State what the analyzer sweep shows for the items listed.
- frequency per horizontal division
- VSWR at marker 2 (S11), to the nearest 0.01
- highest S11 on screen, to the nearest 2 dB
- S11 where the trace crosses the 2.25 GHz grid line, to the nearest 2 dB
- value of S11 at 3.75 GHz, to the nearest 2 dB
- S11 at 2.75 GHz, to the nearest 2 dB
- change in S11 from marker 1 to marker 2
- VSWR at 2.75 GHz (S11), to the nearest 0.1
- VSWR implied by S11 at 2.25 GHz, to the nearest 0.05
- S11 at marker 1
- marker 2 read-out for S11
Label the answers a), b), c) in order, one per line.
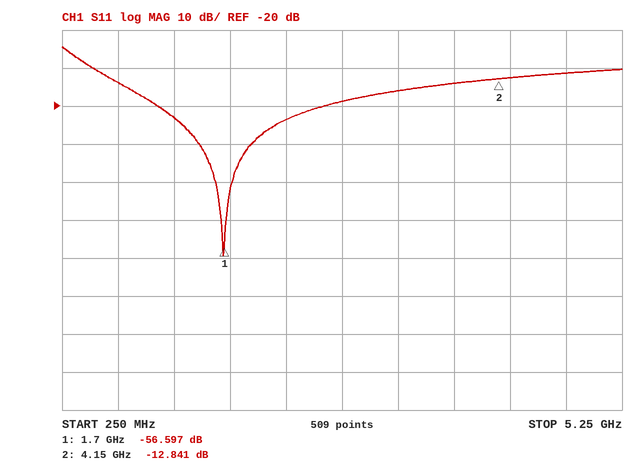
a) 500 MHz
b) 1.59
c) -4 dB
d) -24 dB
e) -14 dB
f) -18 dB
g) 43.756 dB
h) 1.3
i) 1.15
j) -56.597 dB
k) -12.841 dB
